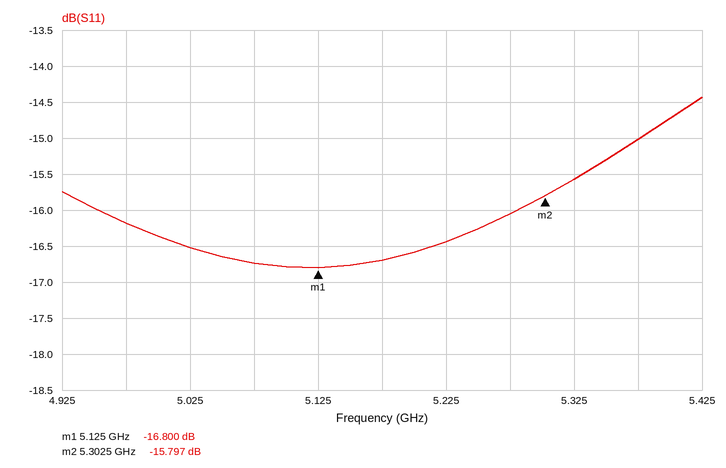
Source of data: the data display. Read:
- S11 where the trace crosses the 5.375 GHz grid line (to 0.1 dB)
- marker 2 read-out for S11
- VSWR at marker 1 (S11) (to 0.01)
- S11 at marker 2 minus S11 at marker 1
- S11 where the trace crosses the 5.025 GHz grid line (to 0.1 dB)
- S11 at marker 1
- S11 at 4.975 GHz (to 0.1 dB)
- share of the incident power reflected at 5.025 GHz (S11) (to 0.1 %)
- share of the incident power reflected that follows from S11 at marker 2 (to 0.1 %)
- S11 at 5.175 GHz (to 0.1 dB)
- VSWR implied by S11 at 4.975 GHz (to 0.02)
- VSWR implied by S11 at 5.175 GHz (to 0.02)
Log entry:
-15.0 dB
-15.797 dB
1.34
1.003 dB
-16.5 dB
-16.800 dB
-16.2 dB
2.2 %
2.6 %
-16.7 dB
1.36
1.34
